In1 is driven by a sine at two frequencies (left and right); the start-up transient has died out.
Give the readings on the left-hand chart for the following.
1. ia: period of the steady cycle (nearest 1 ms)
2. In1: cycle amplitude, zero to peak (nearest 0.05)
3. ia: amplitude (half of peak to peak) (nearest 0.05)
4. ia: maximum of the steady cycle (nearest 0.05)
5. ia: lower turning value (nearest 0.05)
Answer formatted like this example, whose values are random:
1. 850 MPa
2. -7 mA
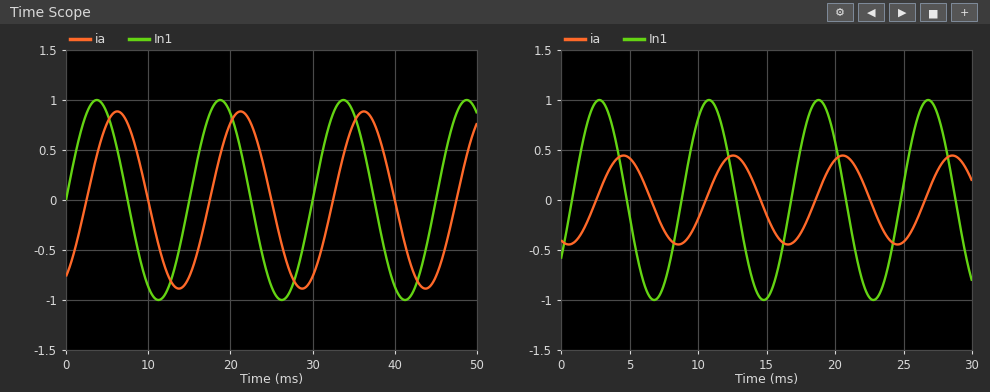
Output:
1. 15 ms
2. 1.00
3. 0.90
4. 0.90
5. -0.90
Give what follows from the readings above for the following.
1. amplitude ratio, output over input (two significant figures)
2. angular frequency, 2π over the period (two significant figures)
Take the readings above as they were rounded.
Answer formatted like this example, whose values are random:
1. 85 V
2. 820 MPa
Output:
1. 0.90
2. 0.42 rad/ms
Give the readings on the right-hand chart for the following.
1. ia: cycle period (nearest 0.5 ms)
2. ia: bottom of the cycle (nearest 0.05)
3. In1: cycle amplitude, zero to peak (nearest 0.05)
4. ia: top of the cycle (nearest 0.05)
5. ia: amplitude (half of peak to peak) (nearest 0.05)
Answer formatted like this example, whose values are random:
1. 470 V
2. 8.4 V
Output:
1. 8.0 ms
2. -0.45
3. 1.00
4. 0.45
5. 0.45
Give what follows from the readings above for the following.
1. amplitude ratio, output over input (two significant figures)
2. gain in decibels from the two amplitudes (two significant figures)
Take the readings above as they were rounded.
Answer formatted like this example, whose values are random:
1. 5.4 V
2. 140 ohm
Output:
1. 0.45
2. -6.9 dB
